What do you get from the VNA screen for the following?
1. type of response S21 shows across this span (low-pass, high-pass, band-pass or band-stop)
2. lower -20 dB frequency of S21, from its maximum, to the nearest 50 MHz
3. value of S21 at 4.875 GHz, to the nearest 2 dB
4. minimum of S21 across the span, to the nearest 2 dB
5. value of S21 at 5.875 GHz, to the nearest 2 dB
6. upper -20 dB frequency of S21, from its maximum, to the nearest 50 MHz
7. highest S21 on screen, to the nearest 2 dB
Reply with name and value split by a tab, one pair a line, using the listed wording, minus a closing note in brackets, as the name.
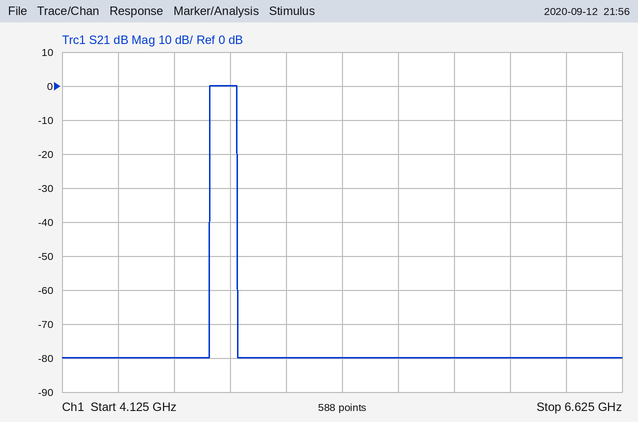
type of response S21 shows across this span	band-pass
lower -20 dB frequency of S21, from its maximum, to the nearest 50 MHz	4.80 GHz
value of S21 at 4.875 GHz, to the nearest 2 dB	0 dB
minimum of S21 across the span, to the nearest 2 dB	-80 dB
value of S21 at 5.875 GHz, to the nearest 2 dB	-80 dB
upper -20 dB frequency of S21, from its maximum, to the nearest 50 MHz	4.90 GHz
highest S21 on screen, to the nearest 2 dB	0 dB
